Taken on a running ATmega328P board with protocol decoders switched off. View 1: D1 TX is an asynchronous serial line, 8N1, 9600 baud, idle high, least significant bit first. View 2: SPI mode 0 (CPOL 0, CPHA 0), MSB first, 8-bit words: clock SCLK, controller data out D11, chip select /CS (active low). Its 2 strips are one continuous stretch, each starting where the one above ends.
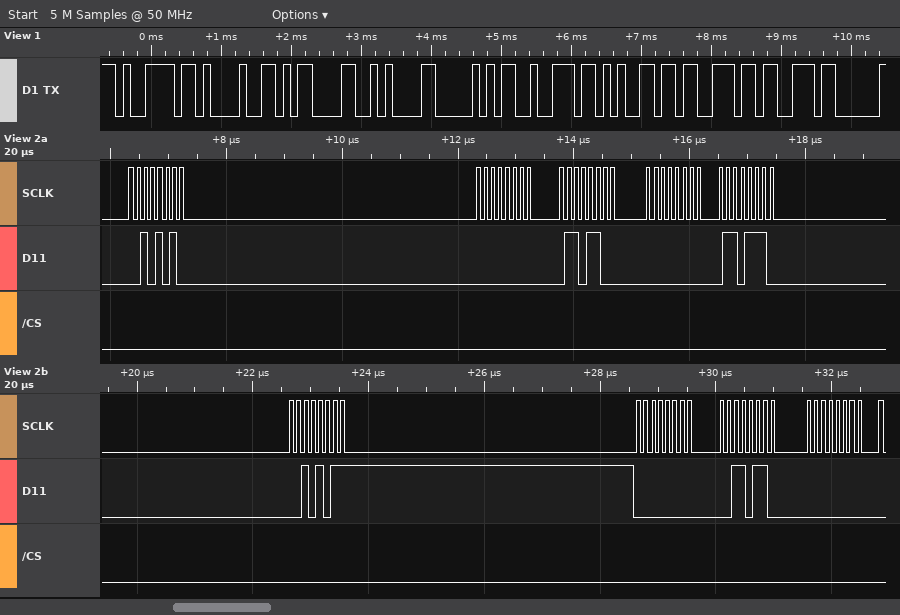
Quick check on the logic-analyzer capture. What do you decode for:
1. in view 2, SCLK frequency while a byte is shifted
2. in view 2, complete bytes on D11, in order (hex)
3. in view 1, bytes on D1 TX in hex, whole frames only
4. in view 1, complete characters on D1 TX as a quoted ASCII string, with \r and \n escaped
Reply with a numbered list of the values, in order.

1. 8 MHz
2. 2A 00 6C 00 6E 2B 00 36 00
3. 79 21 0D 0A 50 72 65 73 73
4. "y!\r\nPress"
